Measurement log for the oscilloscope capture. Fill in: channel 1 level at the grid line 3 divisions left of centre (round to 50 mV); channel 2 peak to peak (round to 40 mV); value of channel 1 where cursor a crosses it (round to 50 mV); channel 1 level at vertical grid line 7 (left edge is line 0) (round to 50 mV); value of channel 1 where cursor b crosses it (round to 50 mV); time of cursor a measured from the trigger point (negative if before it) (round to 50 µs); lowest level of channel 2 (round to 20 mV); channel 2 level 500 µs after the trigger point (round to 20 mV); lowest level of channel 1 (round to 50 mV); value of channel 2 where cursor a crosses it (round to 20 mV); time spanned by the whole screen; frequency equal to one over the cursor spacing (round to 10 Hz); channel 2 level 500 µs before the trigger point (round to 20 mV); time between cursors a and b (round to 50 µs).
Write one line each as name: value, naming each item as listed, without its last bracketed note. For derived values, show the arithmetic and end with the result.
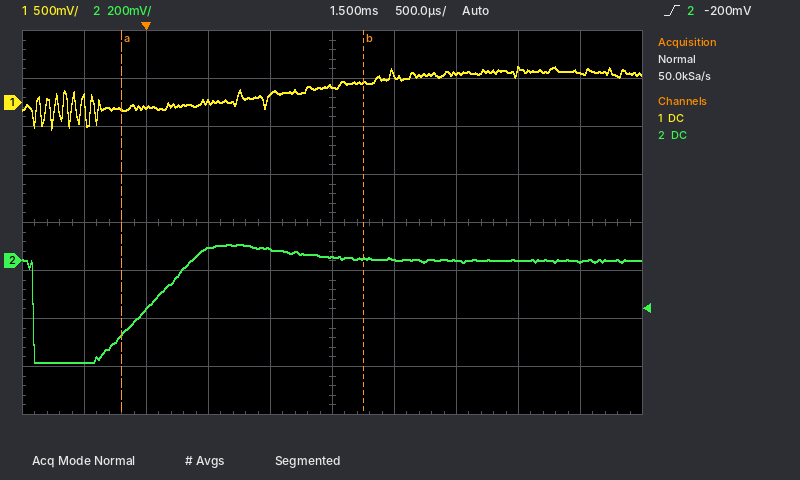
channel 1 level at the grid line 3 divisions left of centre: -50 mV
channel 2 peak to peak: 480 mV
value of channel 1 where cursor a crosses it: -50 mV
channel 1 level at vertical grid line 7 (left edge is line 0): 300 mV
value of channel 1 where cursor b crosses it: 200 mV
time of cursor a measured from the trigger point (negative if before it): -200 µs
lowest level of channel 2: -420 mV
channel 2 level 500 µs after the trigger point: 60 mV
lowest level of channel 1: -300 mV
value of channel 2 where cursor a crosses it: -300 mV
time spanned by the whole screen: 5 ms
frequency equal to one over the cursor spacing: 1 / 1.95 ms ≈ 510 Hz
channel 2 level 500 µs before the trigger point: -420 mV
time between cursors a and b: 1.95 ms
